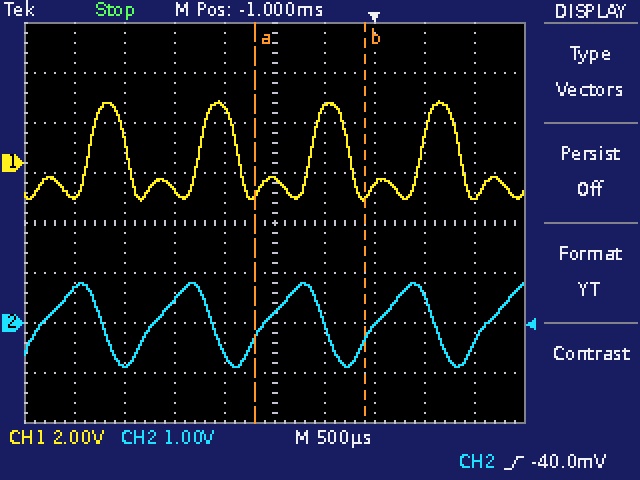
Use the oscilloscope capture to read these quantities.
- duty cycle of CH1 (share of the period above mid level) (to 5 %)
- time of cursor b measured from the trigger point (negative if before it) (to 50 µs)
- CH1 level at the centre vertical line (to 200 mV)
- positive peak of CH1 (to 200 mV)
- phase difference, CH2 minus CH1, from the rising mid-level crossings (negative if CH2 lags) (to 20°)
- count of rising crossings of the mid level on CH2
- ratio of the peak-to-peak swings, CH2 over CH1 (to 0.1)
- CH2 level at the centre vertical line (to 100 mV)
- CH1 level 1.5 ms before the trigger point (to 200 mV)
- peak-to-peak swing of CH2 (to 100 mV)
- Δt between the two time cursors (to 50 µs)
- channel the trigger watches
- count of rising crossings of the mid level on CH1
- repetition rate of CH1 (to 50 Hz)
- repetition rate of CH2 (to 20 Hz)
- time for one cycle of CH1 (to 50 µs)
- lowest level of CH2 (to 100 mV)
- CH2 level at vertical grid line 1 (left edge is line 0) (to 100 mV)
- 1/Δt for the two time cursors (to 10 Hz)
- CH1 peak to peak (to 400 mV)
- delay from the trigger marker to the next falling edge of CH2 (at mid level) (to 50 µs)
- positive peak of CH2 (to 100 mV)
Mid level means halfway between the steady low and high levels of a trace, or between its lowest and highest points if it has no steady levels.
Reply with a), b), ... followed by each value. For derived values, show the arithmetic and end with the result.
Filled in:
a) 35 %
b) -100 µs
c) -600 mV
d) 2.4 V
e) +160°
f) 5
g) 1.7 V / 4.0 V ≈ 0.4
h) 200 mV
i) 2.2 V
j) 800 mV − (-900 mV) = 1.7 V
k) 1.10 ms
l) CH2
m) 4
n) 1 / 1.10 ms ≈ 909 Hz, so 900 Hz to the nearest 50 Hz
o) 900 Hz
p) 1.10 ms
q) -900 mV
r) 700 mV
s) 1 / 1.10 ms ≈ 910 Hz
t) 4.0 V
u) 600 µs
v) 800 mV
